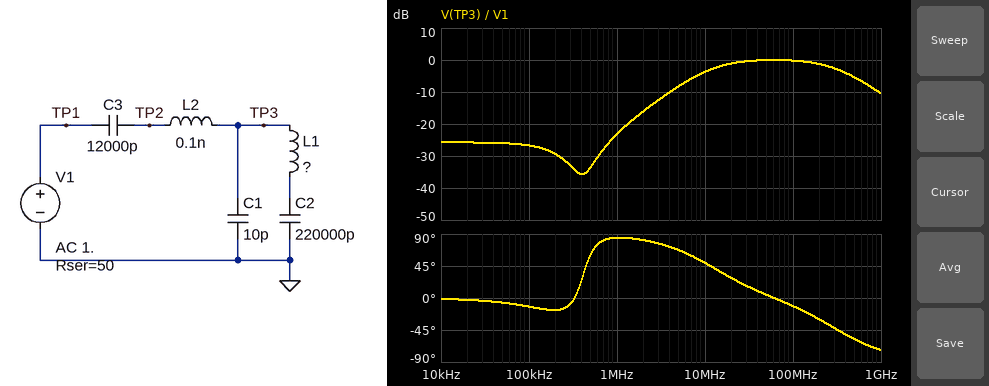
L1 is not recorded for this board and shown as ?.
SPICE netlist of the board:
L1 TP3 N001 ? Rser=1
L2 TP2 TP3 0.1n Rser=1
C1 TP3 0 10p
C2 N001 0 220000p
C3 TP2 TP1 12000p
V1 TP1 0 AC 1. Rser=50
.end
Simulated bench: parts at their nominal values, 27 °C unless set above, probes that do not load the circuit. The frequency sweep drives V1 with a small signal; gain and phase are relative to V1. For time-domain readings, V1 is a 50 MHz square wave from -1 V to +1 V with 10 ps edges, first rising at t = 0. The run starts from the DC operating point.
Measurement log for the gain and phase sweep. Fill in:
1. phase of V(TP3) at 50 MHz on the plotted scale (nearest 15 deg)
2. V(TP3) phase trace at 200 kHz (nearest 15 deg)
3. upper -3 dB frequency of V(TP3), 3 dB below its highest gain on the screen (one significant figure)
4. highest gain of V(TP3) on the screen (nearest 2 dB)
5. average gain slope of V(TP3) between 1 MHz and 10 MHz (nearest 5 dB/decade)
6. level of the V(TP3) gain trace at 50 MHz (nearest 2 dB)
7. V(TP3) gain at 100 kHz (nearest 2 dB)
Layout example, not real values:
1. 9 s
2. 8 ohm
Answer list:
1. 0 deg
2. -15 deg
3. 300 MHz
4. 0 dB
5. 20 dB/decade
6. 0 dB
7. -26 dB
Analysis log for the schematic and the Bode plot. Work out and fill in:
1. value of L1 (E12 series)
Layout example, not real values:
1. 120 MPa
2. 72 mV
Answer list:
1. 680 nH
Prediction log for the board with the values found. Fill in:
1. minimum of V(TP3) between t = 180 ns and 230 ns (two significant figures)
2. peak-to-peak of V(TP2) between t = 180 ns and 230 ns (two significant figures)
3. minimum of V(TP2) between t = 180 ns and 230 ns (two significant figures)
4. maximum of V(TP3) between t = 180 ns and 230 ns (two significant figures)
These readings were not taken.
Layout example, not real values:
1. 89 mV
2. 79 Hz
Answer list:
1. -1.2 V
2. 2.4 V
3. -1.2 V
4. 1.2 V
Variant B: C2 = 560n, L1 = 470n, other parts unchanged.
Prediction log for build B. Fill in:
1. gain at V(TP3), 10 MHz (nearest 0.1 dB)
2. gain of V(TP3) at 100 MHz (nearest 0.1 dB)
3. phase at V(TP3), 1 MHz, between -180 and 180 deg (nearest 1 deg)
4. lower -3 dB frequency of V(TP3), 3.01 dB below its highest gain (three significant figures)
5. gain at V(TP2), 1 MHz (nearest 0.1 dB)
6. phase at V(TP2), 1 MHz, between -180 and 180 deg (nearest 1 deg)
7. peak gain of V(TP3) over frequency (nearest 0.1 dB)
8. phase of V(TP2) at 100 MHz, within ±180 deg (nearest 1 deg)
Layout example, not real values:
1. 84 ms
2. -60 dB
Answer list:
1. -5.9 dB
2. -0.1 dB
3. 81 deg
4. 16.5 MHz
5. -24.0 dB
6. 65 deg
7. 0 dB
8. -8 deg
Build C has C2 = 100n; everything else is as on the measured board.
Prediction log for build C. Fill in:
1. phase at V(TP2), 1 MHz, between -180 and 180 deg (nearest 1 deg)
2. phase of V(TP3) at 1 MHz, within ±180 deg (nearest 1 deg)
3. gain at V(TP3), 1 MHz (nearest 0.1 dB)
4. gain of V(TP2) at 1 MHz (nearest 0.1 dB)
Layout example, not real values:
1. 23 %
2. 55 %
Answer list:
1. 65 deg
2. 81 deg
3. -25.4 dB
4. -24.0 dB
